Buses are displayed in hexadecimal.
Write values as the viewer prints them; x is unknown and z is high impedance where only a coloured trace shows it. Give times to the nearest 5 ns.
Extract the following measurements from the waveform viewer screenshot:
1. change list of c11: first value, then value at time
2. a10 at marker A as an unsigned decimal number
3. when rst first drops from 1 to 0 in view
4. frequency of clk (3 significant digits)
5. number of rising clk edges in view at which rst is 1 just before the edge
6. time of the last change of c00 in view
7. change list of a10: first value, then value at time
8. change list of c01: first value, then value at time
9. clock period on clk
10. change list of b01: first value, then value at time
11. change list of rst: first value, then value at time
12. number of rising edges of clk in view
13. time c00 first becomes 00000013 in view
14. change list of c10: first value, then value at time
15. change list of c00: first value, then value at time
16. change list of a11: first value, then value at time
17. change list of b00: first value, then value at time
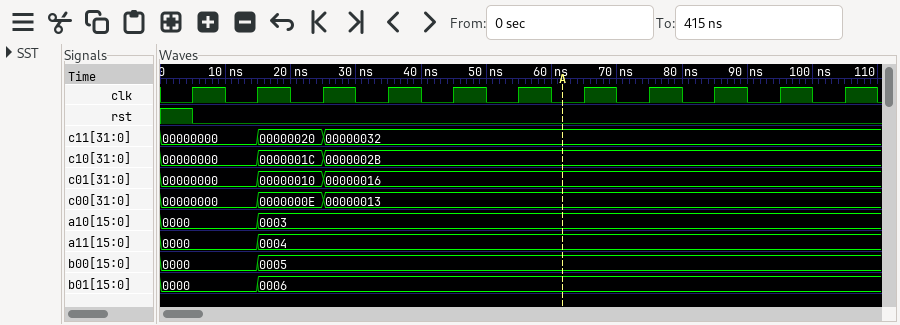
00000000, 00000020 at 15 ns, 00000032 at 25 ns
3
5 ns
100 MHz
1
25 ns
0000, 0003 at 15 ns
00000000, 00000010 at 15 ns, 00000016 at 25 ns
10 ns
0000, 0006 at 15 ns
1, 0 at 5 ns
11
25 ns
00000000, 0000001C at 15 ns, 0000002B at 25 ns
00000000, 0000000E at 15 ns, 00000013 at 25 ns
0000, 0004 at 15 ns
0000, 0005 at 15 ns
